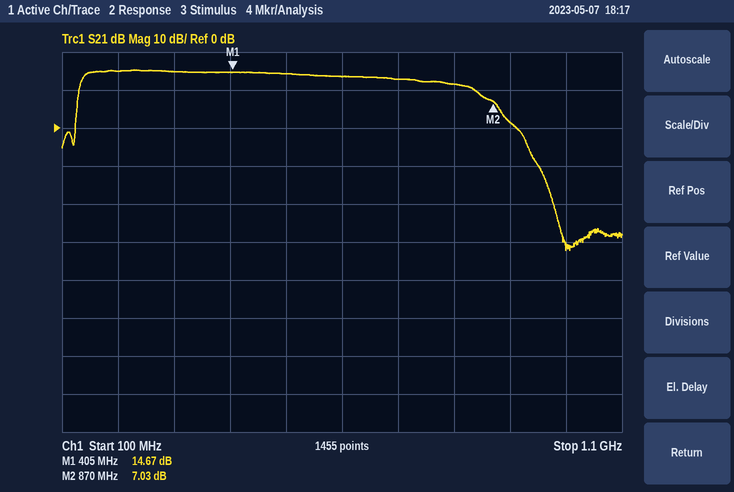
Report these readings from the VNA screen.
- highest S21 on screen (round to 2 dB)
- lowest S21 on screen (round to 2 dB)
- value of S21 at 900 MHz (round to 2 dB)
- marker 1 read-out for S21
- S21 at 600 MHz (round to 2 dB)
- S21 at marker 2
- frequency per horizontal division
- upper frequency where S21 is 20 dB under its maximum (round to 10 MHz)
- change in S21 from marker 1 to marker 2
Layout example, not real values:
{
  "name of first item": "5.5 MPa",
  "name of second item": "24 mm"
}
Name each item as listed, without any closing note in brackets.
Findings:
{
  "highest S21 on screen": "16 dB",
  "lowest S21 on screen": "-32 dB",
  "value of S21 at 900 MHz": "2 dB",
  "marker 1 read-out for S21": "14.67 dB",
  "S21 at 600 MHz": "14 dB",
  "S21 at marker 2": "7.03 dB",
  "frequency per horizontal division": "100 MHz",
  "upper frequency where S21 is 20 dB under its maximum": "930 MHz",
  "change in S21 from marker 1 to marker 2": "-7.64 dB"
}
